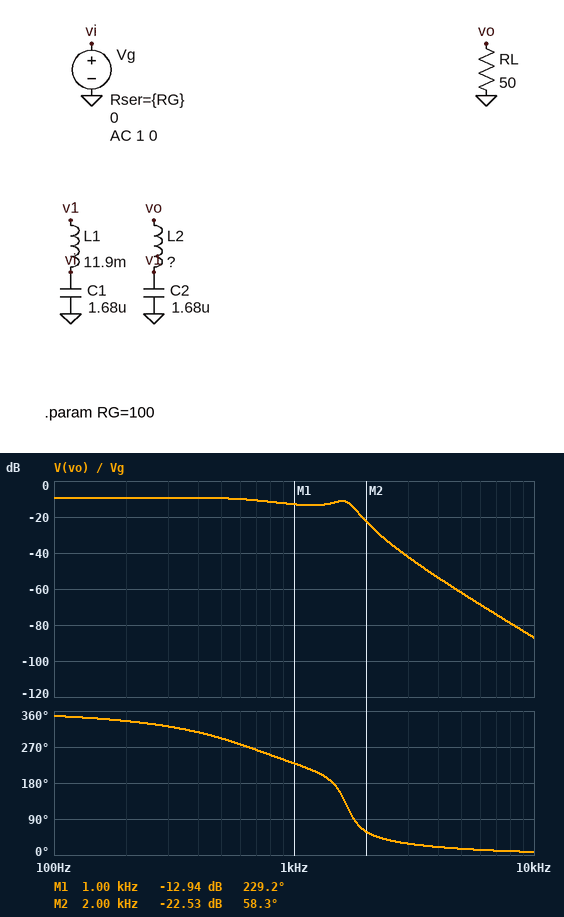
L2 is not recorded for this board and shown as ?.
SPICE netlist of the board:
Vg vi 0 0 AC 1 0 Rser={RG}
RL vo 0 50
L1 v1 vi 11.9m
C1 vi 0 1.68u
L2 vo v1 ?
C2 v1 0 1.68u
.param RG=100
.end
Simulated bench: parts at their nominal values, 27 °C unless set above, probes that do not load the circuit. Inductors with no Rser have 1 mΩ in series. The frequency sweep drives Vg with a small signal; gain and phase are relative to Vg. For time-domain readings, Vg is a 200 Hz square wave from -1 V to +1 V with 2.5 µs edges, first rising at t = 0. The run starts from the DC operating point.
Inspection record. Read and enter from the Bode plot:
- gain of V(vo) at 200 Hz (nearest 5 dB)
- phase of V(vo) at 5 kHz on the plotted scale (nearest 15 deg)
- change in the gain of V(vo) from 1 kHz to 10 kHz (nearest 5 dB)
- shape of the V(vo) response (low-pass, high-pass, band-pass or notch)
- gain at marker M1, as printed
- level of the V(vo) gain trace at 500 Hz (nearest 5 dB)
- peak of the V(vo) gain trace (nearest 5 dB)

-10 dB
15 deg
-75 dB
low-pass
-12.94 dB
-10 dB
-10 dB
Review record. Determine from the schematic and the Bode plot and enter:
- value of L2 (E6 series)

22 mH
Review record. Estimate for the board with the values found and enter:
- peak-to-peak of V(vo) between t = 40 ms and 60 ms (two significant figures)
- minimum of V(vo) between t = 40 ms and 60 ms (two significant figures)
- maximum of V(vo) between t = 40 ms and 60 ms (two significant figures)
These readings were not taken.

790 mV
-390 mV
390 mV
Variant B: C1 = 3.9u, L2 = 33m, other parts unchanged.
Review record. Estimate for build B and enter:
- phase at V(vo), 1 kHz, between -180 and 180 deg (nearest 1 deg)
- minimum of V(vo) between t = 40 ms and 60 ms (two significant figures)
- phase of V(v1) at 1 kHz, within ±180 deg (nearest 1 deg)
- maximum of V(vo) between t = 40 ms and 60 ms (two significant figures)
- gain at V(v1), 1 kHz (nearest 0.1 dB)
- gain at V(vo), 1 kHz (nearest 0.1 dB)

-154 deg
-430 mV
-77 deg
430 mV
-6.4 dB
-19.0 dB
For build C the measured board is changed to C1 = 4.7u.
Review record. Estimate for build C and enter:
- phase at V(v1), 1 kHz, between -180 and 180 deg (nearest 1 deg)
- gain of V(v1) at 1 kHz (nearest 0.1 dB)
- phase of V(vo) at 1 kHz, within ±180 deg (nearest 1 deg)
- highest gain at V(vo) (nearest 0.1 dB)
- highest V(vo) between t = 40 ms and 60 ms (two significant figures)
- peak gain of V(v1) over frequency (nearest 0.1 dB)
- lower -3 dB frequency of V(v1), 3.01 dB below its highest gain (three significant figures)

-81 deg
-8.5 dB
-151 deg
-9.0 dB
430 mV
3.1 dB
1.41 kHz
